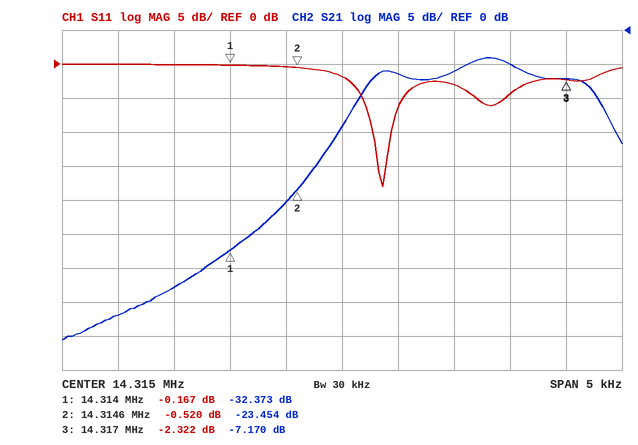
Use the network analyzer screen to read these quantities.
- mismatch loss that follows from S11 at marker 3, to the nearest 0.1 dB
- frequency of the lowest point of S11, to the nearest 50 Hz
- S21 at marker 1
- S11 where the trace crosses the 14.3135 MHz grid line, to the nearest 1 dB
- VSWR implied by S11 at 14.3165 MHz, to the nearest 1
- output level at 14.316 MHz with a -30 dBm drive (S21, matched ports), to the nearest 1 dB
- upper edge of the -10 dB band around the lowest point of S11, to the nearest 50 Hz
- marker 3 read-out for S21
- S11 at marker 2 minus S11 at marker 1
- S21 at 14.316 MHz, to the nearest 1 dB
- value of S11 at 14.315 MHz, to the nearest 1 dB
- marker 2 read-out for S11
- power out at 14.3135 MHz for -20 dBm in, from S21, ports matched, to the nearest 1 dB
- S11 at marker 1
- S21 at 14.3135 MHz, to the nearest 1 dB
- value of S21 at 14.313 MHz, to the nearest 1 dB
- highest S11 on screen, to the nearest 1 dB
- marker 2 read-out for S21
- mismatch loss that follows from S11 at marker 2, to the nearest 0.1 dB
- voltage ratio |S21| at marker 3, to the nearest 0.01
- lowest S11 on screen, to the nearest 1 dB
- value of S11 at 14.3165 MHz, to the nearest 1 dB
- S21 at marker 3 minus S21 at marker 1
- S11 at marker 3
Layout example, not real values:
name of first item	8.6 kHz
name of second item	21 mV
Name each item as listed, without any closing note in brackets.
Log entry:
mismatch loss that follows from S11 at marker 3, to the nearest 0.1 dB	3.8 dB
frequency of the lowest point of S11, to the nearest 50 Hz	14.31535 MHz
S21 at marker 1	-32.373 dB
S11 where the trace crosses the 14.3135 MHz grid line, to the nearest 1 dB	0 dB
VSWR implied by S11 at 14.3165 MHz, to the nearest 1	4
output level at 14.316 MHz with a -30 dBm drive (S21, matched ports), to the nearest 1 dB	-36 dBm
upper edge of the -10 dB band around the lowest point of S11, to the nearest 50 Hz	14.31545 MHz
marker 3 read-out for S21	-7.170 dB
S11 at marker 2 minus S11 at marker 1	-0.353 dB
S21 at 14.316 MHz, to the nearest 1 dB	-6 dB
value of S11 at 14.315 MHz, to the nearest 1 dB	-2 dB
marker 2 read-out for S11	-0.520 dB
power out at 14.3135 MHz for -20 dBm in, from S21, ports matched, to the nearest 1 dB	-58 dBm
S11 at marker 1	-0.167 dB
S21 at 14.3135 MHz, to the nearest 1 dB	-38 dB
value of S21 at 14.313 MHz, to the nearest 1 dB	-42 dB
highest S11 on screen, to the nearest 1 dB	0 dB
marker 2 read-out for S21	-23.454 dB
mismatch loss that follows from S11 at marker 2, to the nearest 0.1 dB	9.5 dB
voltage ratio |S21| at marker 3, to the nearest 0.01	0.44
lowest S11 on screen, to the nearest 1 dB	-18 dB
value of S11 at 14.3165 MHz, to the nearest 1 dB	-4 dB
S21 at marker 3 minus S21 at marker 1	25.203 dB
S11 at marker 3	-2.322 dB
